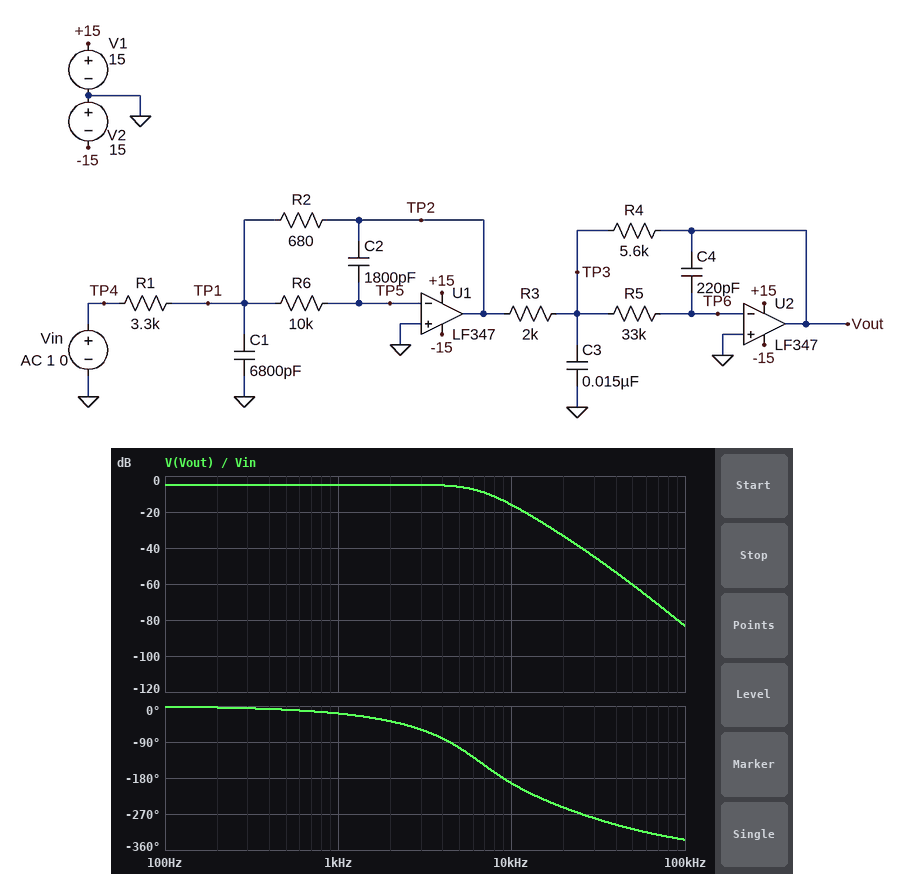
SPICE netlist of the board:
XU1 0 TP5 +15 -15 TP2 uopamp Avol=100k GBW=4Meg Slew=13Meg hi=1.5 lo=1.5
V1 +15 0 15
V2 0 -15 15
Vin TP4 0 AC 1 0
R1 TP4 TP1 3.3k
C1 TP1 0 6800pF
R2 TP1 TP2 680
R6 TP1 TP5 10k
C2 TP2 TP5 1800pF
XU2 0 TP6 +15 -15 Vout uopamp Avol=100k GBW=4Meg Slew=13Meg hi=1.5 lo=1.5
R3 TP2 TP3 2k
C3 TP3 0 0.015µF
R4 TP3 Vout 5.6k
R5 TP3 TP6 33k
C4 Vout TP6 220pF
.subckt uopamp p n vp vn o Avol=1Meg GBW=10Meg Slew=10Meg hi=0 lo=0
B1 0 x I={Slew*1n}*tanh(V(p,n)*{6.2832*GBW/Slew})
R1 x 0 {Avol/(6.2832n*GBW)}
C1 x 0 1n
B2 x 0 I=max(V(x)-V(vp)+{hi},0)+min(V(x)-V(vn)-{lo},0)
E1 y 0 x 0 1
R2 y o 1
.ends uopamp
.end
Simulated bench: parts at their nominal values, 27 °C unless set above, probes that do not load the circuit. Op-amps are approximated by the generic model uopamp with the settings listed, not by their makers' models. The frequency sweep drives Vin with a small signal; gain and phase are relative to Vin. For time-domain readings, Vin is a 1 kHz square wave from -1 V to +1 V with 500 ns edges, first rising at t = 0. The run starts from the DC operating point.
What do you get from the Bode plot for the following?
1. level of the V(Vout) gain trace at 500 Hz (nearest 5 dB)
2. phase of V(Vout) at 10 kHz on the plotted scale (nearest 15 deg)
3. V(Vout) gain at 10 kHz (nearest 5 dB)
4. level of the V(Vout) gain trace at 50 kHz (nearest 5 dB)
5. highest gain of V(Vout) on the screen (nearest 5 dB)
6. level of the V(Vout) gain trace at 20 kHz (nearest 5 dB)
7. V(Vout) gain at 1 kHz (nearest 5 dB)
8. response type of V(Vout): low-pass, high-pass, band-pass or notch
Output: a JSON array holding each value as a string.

["-5 dB", "-195 deg", "-15 dB", "-60 dB", "-5 dB", "-35 dB", "-5 dB", "low-pass"]
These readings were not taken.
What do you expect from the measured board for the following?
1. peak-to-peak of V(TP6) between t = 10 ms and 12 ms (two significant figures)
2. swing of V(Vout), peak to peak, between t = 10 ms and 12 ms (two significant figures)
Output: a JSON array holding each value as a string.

["1.5 mV", "1.3 V"]
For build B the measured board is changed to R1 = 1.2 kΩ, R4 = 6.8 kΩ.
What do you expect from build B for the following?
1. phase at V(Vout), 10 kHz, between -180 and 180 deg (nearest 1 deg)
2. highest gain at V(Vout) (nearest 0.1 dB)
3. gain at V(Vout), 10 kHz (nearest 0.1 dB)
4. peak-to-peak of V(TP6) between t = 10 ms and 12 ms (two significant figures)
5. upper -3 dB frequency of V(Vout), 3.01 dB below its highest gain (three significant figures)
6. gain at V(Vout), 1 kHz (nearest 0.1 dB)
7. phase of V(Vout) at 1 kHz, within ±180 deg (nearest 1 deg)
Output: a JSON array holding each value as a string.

["157 deg", "5.7 dB", "-9.3 dB", "4.1 mV", "4.99 kHz", "5.6 dB", "-23 deg"]
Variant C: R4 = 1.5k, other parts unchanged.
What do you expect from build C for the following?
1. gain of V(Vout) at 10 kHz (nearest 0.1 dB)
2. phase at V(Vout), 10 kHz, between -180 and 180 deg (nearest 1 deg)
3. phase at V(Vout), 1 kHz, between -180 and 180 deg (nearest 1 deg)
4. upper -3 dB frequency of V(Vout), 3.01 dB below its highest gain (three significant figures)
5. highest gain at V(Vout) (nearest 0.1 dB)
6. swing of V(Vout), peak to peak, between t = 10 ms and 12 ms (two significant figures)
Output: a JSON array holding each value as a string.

["-19.3 dB", "-132 deg", "-13 deg", "9.96 kHz", "-16.2 dB", "320 mV"]
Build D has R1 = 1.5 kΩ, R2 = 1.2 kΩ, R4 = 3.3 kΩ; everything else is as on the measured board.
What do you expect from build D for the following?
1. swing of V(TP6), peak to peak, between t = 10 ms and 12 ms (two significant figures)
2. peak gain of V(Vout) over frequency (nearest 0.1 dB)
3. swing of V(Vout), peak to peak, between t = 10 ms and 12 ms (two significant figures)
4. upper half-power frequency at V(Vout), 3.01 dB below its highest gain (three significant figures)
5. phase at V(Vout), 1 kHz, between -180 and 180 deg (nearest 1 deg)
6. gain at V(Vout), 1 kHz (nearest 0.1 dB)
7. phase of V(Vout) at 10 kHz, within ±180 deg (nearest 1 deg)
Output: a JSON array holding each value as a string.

["3.6 mV", "2.4 dB", "2.7 V", "6.27 kHz", "-20 deg", "2.3 dB", "172 deg"]
